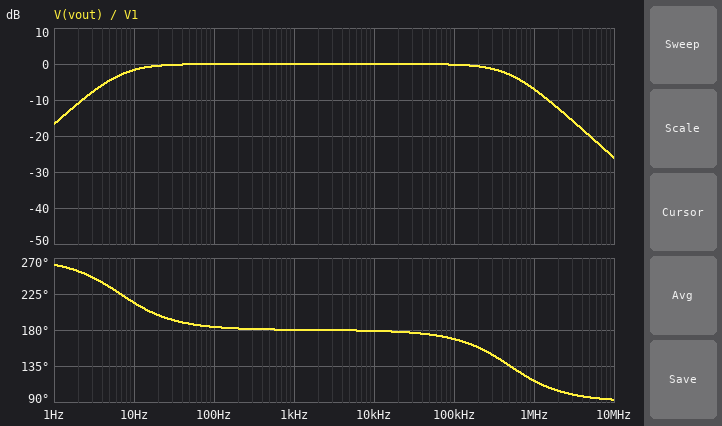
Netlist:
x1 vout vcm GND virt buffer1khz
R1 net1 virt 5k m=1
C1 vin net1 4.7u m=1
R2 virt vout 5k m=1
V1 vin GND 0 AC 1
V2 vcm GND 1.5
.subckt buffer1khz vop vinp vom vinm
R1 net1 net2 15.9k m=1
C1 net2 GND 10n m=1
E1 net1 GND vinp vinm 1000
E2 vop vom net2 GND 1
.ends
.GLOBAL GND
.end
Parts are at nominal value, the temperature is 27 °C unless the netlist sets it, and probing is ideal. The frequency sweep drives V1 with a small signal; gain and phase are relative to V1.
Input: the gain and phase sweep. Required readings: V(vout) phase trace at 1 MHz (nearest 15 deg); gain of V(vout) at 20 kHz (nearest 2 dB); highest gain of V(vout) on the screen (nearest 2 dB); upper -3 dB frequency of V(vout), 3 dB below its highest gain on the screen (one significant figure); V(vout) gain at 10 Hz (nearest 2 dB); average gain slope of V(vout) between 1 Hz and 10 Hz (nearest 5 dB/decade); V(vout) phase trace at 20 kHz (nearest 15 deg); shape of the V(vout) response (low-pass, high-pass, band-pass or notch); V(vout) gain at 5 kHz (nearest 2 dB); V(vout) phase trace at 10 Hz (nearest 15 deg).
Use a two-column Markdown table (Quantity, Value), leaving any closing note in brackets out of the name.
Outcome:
| Quantity | Value |
|---|---|
| V(vout) phase trace at 1 MHz | 120 deg |
| gain of V(vout) at 20 kHz | 0 dB |
| highest gain of V(vout) on the screen | 0 dB |
| upper -3 dB frequency of V(vout), 3 dB below its highest gain on the screen | 500 kHz |
| V(vout) gain at 10 Hz | -2 dB |
| average gain slope of V(vout) between 1 Hz and 10 Hz | 15 dB/decade |
| V(vout) phase trace at 20 kHz | 180 deg |
| shape of the V(vout) response | band-pass |
| V(vout) gain at 5 kHz | 0 dB |
| V(vout) phase trace at 10 Hz | 210 deg |
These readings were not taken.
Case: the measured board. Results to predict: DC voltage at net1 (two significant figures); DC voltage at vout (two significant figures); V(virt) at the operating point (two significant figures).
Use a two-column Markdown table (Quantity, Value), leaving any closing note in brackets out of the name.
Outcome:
| Quantity | Value |
|---|---|
| DC voltage at net1 | 1.5 V |
| DC voltage at vout | 1.5 V |
| V(virt) at the operating point | 1.5 V |
